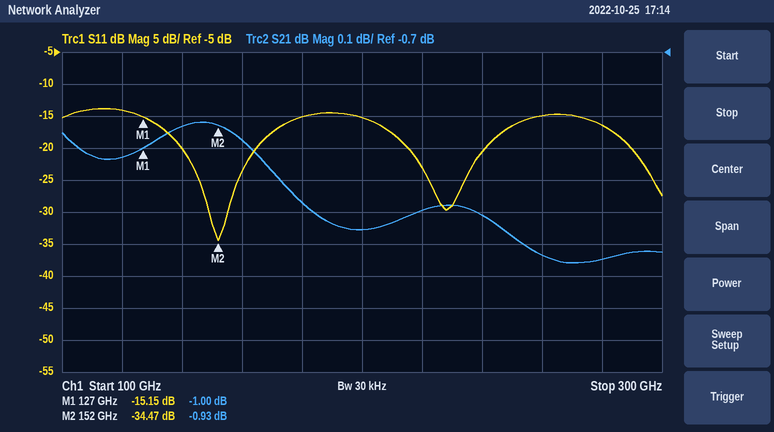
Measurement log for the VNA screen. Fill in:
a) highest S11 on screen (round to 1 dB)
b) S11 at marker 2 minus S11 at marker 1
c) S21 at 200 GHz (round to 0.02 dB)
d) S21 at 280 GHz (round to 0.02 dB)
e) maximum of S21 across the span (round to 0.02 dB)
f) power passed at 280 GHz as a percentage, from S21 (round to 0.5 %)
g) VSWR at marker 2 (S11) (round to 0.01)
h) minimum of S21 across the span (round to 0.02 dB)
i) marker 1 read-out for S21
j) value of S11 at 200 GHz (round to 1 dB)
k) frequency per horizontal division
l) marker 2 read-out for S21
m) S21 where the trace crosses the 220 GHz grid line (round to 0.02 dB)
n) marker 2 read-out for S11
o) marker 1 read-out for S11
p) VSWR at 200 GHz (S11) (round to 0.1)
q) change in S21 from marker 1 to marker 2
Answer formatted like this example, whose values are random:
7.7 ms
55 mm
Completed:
-14 dB
-19.32 dB
-1.26 dB
-1.34 dB
-0.92 dB
73.5 %
1.04
-1.36 dB
-1.00 dB
-15 dB
20 GHz
-0.93 dB
-1.20 dB
-34.47 dB
-15.15 dB
1.4
0.07 dB
